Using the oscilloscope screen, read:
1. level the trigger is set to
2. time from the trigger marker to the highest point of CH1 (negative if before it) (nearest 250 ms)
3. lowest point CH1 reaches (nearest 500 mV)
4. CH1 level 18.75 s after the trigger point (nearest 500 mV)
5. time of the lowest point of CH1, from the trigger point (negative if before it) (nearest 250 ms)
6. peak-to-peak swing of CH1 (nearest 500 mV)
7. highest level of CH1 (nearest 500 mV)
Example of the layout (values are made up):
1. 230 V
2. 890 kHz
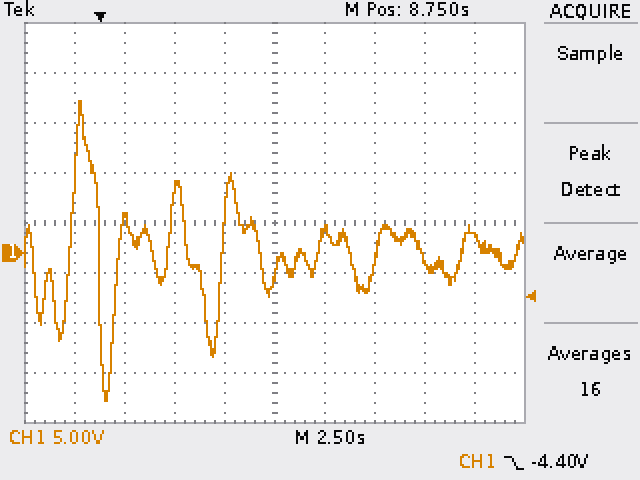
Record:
1. -4.40 V
2. -1.00 s
3. -15.0 V
4. 1.5 V
5. +250 ms
6. 30.0 V
7. 15.0 V
